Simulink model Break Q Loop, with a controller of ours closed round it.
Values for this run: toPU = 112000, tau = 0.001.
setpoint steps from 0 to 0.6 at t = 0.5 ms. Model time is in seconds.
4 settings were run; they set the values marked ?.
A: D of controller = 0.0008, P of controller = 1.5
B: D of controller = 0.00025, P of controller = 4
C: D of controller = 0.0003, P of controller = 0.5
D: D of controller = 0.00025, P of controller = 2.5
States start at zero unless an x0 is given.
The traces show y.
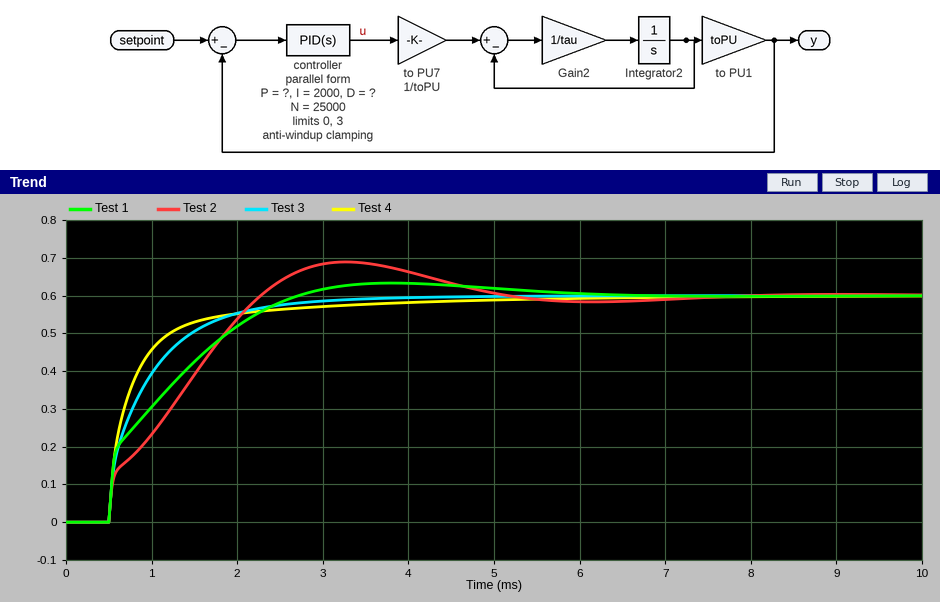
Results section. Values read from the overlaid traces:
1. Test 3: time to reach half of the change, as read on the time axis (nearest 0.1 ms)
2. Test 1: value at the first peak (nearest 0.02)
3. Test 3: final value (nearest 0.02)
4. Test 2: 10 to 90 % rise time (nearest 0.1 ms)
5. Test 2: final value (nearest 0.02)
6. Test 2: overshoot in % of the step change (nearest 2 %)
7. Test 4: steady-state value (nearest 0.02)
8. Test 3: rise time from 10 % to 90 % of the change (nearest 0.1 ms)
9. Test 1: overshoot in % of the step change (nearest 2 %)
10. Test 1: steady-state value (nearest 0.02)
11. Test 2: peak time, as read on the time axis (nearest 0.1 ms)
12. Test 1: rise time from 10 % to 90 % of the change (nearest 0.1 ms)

0.8 ms
0.64
0.60
1.5 ms
0.60
14 %
0.60
1.3 ms
6 %
0.60
3.3 ms
1.6 ms
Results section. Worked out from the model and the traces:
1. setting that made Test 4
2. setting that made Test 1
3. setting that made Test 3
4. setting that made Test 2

B
A
D
C
